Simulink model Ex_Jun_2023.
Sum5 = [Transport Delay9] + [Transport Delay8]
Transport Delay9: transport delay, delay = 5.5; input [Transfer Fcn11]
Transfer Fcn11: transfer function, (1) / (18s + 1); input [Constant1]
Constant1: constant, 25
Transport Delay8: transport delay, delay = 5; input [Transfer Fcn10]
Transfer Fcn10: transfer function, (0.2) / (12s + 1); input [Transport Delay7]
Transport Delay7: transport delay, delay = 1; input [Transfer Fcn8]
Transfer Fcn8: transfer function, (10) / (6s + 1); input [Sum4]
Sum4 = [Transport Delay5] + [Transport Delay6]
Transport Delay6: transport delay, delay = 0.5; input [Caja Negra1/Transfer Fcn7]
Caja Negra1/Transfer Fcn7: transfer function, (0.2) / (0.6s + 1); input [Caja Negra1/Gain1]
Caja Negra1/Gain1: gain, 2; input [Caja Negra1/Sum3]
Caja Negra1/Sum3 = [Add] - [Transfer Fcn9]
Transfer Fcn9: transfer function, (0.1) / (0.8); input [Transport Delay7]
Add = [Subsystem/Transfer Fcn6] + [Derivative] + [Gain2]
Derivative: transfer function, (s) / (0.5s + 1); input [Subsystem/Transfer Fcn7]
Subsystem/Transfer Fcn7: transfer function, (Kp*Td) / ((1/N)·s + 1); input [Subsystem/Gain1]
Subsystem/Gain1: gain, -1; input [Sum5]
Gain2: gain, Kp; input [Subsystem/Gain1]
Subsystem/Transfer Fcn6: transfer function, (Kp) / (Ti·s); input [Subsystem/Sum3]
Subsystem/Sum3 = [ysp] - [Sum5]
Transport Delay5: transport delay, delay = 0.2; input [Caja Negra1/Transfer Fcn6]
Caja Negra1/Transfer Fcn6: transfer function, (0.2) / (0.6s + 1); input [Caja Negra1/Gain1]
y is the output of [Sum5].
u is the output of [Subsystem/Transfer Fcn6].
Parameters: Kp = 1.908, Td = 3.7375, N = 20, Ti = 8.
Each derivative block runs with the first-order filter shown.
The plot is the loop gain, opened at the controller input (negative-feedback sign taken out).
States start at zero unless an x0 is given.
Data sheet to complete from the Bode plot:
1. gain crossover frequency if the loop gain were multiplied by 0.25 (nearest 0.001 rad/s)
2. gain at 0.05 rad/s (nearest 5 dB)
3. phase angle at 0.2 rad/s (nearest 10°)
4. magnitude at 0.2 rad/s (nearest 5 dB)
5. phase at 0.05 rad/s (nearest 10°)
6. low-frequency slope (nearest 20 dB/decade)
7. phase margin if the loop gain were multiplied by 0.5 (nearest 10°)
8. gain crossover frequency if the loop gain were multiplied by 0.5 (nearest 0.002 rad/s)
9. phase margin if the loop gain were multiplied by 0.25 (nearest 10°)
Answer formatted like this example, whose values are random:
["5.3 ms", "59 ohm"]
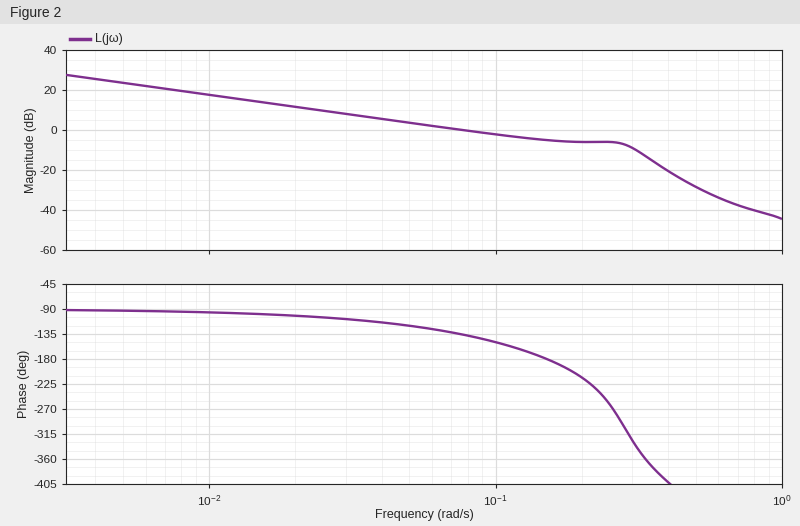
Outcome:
["0.019 rad/s", "5 dB", "-210°", "-5 dB", "-120°", "-20 dB/decade", "70°", "0.038 rad/s", "80°"]
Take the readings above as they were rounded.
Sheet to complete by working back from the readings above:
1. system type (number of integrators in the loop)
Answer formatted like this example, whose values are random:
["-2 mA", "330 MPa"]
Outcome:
["1"]
